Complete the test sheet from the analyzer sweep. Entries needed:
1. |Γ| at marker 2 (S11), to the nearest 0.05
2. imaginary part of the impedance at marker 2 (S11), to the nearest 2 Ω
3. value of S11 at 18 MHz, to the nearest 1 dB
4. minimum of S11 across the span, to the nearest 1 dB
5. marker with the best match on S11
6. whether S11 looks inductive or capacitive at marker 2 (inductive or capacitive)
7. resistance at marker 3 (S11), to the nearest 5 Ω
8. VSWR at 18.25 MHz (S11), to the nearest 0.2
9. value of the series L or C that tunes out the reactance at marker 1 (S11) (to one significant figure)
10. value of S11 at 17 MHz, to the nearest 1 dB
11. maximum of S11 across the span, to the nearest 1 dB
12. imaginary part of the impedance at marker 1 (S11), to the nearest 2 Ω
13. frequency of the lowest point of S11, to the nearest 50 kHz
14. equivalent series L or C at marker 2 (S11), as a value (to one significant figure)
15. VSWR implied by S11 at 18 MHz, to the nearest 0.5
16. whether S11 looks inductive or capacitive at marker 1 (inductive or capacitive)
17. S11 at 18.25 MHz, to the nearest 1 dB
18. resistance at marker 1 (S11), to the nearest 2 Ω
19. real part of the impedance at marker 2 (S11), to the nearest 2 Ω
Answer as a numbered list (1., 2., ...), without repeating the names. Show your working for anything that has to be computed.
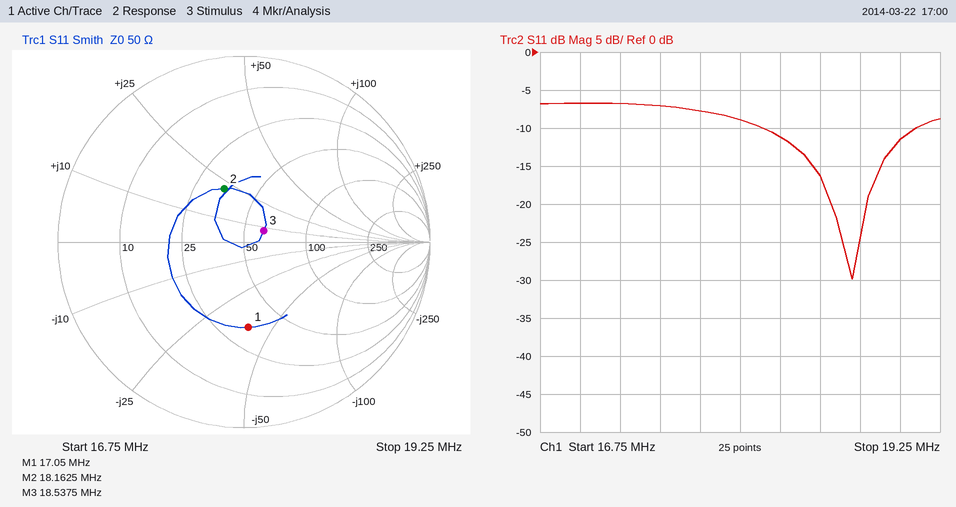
1. 0.30
2. +22 Ω
3. -9 dB
4. -30 dB
5. marker 3
6. inductive
7. 60 Ω
8. |Γ| = 10^(-11/20) = 0.2818; VSWR = (1 + 0.2818)/(1 − 0.2818) ≈ 1.8
9. L = 40 Ω/(2π × 17.05 MHz) ≈ 373 nH, so 400 nH to one significant figure
10. -7 dB
11. -7 dB
12. -40 Ω
13. 18.70 MHz
14. L = 22 Ω/(2π × 18.1625 MHz) ≈ 193 nH, so 200 nH to one significant figure
15. |Γ| = 10^(-9/20) = 0.3548; VSWR = (1 + 0.3548)/(1 − 0.3548) ≈ 2.10, so 2.0 to the nearest 0.5
16. capacitive
17. -11 dB
18. 34 Ω
19. 34 Ω
